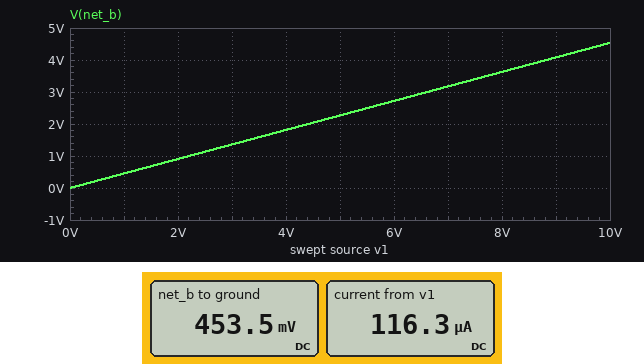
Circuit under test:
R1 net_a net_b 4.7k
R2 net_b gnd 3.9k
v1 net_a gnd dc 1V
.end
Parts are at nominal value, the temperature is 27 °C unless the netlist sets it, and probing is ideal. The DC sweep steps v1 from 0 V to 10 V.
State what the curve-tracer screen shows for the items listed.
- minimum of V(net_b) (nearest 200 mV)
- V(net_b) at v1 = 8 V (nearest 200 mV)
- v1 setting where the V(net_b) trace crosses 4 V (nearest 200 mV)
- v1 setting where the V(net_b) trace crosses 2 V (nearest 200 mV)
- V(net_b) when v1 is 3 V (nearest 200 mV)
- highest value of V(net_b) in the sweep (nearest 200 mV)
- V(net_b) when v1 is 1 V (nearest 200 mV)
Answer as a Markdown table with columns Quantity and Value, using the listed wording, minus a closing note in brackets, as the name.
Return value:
| Quantity | Value |
|---|---|
| minimum of V(net_b) | 0 V |
| V(net_b) at v1 = 8 V | 3.6 V |
| v1 setting where the V(net_b) trace crosses 4 V | 8.8 V |
| v1 setting where the V(net_b) trace crosses 2 V | 4.4 V |
| V(net_b) when v1 is 3 V | 1.4 V |
| highest value of V(net_b) in the sweep | 4.6 V |
| V(net_b) when v1 is 1 V | 400 mV |
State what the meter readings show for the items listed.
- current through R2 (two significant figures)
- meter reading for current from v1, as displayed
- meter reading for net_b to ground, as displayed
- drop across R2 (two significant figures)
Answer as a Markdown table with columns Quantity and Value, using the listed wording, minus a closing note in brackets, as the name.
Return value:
| Quantity | Value |
|---|---|
| current through R2 | 120 µA |
| meter reading for current from v1, as displayed | 116.3 µA |
| meter reading for net_b to ground, as displayed | 453.5 mV |
| drop across R2 | 450 mV |
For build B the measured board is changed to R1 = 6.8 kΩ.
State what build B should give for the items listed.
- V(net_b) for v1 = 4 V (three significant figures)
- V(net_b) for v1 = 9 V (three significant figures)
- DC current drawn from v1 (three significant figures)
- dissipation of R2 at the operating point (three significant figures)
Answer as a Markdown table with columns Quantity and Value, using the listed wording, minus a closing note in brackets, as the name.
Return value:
| Quantity | Value |
|---|---|
| V(net_b) for v1 = 4 V | 1.46 V |
| V(net_b) for v1 = 9 V | 3.28 V |
| DC current drawn from v1 | 93.5 µA |
| dissipation of R2 at the operating point | 34.1 µW |
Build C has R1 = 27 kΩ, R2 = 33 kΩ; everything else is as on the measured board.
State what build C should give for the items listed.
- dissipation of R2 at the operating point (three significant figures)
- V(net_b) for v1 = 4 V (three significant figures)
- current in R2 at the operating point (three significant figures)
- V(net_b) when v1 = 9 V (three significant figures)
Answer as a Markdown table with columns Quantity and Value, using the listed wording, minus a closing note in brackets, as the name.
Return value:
| Quantity | Value |
|---|---|
| dissipation of R2 at the operating point | 9.17 µW |
| V(net_b) for v1 = 4 V | 2.20 V |
| current in R2 at the operating point | 16.7 µA |
| V(net_b) when v1 = 9 V | 4.95 V |
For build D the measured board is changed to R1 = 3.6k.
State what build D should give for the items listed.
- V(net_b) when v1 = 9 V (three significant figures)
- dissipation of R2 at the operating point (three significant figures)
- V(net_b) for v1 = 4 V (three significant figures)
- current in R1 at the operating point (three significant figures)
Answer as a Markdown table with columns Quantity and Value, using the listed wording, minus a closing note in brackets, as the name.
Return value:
| Quantity | Value |
|---|---|
| V(net_b) when v1 = 9 V | 4.68 V |
| dissipation of R2 at the operating point | 69.3 µW |
| V(net_b) for v1 = 4 V | 2.08 V |
| current in R1 at the operating point | 133 µA |
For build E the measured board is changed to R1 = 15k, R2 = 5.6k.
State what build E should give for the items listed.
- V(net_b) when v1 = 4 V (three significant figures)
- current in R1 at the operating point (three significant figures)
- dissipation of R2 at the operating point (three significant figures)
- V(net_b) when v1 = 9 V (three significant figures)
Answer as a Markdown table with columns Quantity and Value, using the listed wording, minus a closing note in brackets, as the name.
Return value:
| Quantity | Value |
|---|---|
| V(net_b) when v1 = 4 V | 1.09 V |
| current in R1 at the operating point | 48.5 µA |
| dissipation of R2 at the operating point | 13.2 µW |
| V(net_b) when v1 = 9 V | 2.45 V |
